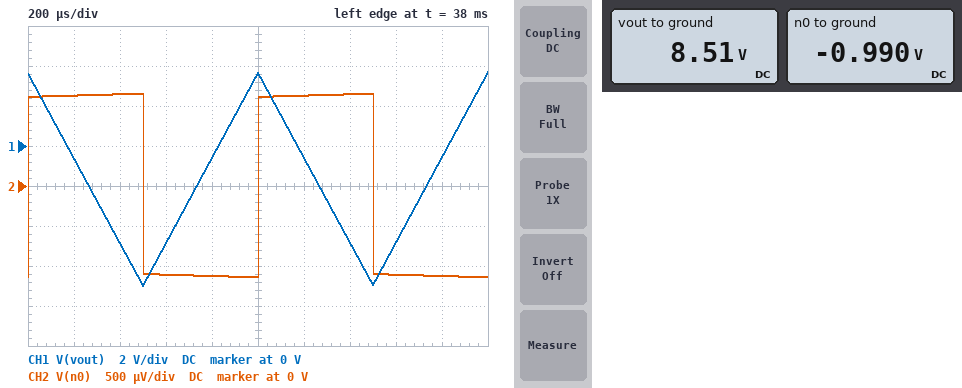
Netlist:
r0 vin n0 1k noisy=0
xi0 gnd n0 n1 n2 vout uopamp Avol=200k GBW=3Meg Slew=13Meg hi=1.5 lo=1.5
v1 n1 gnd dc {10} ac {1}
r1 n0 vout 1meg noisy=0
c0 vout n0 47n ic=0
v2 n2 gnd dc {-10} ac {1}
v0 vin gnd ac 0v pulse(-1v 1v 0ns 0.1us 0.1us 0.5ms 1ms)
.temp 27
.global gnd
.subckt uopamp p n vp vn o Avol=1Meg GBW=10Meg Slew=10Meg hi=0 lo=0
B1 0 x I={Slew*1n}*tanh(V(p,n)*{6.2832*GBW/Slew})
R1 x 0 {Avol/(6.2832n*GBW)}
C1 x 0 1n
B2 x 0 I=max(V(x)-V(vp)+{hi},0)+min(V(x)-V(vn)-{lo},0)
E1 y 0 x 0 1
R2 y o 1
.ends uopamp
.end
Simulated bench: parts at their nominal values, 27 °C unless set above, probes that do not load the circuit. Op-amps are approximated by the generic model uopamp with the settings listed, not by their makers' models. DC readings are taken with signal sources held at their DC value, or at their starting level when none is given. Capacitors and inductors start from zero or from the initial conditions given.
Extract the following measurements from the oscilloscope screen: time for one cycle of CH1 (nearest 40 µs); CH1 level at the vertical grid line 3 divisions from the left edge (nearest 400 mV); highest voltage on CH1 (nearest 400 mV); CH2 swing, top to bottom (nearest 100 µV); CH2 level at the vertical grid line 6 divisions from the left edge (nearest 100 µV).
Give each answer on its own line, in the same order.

1.00 ms
-4.8 V
3.6 V
2.3 mV
1.1 mV
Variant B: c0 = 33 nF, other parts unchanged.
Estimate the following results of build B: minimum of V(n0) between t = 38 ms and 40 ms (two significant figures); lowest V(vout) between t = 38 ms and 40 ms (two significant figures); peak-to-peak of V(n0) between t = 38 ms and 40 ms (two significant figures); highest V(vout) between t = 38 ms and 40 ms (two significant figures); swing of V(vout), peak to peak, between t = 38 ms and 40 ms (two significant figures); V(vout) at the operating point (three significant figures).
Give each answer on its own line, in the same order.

-1.6 mV
-8.1 V
3.3 mV
7.1 V
15 V
8.51 V
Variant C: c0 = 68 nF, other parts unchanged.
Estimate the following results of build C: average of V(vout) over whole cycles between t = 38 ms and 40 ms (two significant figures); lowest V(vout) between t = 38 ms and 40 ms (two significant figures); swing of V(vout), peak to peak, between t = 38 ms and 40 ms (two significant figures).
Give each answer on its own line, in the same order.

-2.2 V
-5.8 V
7.4 V
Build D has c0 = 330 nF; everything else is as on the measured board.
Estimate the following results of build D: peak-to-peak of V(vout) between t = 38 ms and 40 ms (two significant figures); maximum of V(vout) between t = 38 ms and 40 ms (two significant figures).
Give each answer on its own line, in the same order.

1.5 V
65 mV
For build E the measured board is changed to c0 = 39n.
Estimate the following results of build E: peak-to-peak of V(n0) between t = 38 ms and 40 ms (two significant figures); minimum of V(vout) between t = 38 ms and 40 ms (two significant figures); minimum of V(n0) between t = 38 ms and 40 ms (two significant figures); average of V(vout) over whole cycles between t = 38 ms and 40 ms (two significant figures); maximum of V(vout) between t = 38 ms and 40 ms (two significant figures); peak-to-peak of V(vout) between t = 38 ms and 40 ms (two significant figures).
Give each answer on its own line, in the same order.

2.8 mV
-7.4 V
-1.4 mV
-1.0 V
5.4 V
13 V
